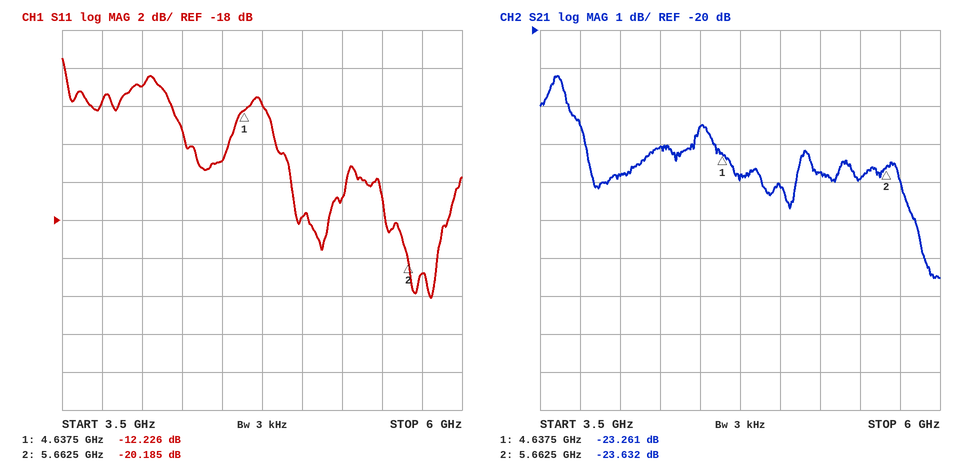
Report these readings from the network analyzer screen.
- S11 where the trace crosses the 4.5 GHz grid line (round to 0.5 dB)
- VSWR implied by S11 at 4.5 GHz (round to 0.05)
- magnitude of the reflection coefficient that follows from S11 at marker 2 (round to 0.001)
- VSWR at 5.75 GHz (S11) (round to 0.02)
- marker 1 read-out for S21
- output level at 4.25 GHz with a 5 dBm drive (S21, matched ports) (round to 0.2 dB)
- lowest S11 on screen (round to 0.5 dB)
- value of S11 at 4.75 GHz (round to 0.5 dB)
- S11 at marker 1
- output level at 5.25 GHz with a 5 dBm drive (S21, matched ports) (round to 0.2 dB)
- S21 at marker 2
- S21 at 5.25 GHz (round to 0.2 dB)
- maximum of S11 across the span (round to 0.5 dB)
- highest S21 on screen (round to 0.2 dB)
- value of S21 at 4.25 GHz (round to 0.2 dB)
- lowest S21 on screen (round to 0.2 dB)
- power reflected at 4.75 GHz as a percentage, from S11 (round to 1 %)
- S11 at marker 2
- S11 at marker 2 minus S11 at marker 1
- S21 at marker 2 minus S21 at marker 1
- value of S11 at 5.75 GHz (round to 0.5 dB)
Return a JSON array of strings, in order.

["-15.0 dB", "1.45", "0.098", "1.20", "-23.261 dB", "-18.0 dBm", "-22.0 dB", "-12.0 dB", "-12.226 dB", "-18.8 dBm", "-23.632 dB", "-23.8 dB", "-9.5 dB", "-21.2 dB", "-23.0 dB", "-26.6 dB", "6 %", "-20.185 dB", "-7.959 dB", "-0.371 dB", "-21.0 dB"]
